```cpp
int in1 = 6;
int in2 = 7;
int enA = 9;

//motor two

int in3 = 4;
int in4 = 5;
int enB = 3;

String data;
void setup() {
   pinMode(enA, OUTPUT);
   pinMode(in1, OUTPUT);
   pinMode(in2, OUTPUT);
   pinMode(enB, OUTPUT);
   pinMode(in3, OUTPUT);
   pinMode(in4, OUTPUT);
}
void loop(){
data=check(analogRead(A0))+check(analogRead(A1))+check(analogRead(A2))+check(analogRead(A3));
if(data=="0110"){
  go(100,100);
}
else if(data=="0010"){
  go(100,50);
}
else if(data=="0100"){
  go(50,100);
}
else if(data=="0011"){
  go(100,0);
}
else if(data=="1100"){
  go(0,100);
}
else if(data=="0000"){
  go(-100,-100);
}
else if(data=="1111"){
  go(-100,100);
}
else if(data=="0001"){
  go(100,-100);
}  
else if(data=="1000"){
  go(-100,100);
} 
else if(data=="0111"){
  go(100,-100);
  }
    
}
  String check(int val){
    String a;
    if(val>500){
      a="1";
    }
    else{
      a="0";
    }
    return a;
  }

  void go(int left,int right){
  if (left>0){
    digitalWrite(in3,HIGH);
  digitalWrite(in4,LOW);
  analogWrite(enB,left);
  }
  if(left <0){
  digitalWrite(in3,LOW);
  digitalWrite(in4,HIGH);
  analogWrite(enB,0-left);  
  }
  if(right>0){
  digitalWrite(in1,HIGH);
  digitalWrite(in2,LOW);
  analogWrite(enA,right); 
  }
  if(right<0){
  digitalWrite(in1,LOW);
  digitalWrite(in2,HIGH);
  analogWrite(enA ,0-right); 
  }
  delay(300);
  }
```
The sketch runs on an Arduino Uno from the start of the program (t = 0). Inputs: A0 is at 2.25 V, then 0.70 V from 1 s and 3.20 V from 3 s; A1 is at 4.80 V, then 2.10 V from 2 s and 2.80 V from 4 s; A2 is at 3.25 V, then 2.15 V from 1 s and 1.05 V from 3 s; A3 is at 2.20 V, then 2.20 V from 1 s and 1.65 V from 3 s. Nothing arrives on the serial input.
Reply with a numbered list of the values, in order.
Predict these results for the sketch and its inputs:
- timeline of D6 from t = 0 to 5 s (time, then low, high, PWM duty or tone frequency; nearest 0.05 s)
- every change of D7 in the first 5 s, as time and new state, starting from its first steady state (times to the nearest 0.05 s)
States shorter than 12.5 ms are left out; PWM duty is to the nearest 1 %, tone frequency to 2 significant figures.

1. 0 s high; 2.1 s low; 3 s high
2. 0 s low; 2.1 s high; 3 s low
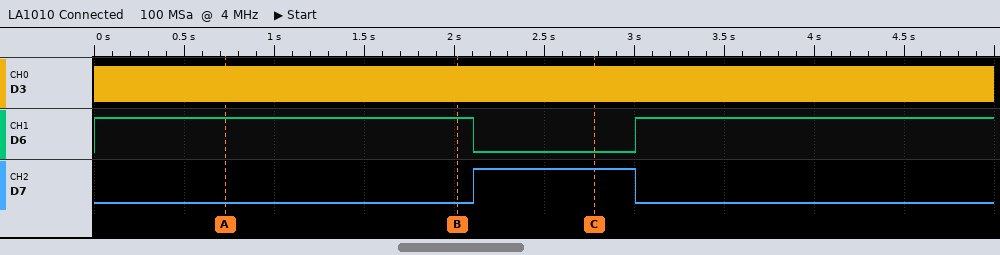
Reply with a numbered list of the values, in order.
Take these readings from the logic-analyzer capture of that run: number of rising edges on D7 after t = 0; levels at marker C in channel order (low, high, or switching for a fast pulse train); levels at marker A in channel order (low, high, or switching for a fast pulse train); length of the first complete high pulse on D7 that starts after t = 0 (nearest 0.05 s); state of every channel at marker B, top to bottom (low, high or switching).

1. 1
2. D3 switching, D6 low, D7 high
3. D3 switching, D6 high, D7 low
4. 0.90 s
5. D3 switching, D6 high, D7 low
